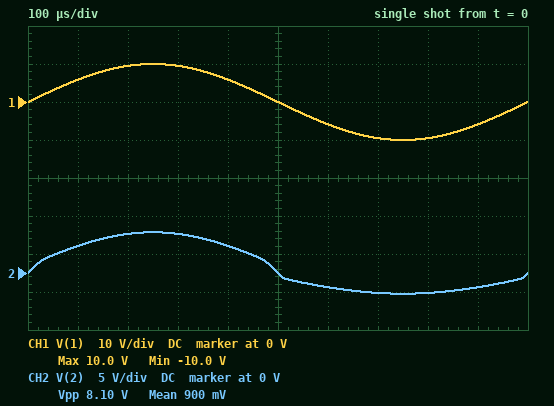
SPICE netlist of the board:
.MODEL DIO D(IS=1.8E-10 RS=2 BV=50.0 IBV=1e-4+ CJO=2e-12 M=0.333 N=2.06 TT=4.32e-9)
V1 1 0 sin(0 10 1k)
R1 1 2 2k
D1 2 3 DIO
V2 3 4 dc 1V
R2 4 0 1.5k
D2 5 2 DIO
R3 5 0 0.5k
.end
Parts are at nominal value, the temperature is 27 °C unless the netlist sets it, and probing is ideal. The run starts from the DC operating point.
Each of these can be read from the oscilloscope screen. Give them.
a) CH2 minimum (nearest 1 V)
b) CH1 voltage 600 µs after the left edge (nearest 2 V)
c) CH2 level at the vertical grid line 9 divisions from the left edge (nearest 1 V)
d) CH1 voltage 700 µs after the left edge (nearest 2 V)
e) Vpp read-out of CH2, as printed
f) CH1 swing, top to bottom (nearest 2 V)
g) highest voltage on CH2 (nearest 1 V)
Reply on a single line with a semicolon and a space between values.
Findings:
-3 V; -6 V; -2 V; -10 V; 8.10 V; 20 V; 5 V
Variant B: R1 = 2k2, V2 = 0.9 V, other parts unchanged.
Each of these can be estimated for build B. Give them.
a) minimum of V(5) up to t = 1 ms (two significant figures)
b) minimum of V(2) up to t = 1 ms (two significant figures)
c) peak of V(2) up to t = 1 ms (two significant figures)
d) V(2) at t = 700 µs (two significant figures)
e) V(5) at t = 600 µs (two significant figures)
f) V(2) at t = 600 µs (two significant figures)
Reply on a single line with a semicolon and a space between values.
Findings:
-1.7 V; -2.6 V; 5.1 V; -2.5 V; -930 mV; -1.8 V
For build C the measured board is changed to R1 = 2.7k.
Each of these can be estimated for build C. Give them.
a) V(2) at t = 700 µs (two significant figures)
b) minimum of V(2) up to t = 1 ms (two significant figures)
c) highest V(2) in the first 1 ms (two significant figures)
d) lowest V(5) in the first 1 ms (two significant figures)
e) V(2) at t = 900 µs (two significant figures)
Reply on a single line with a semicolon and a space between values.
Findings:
-2.2 V; -2.3 V; 4.8 V; -1.4 V; -1.6 V
